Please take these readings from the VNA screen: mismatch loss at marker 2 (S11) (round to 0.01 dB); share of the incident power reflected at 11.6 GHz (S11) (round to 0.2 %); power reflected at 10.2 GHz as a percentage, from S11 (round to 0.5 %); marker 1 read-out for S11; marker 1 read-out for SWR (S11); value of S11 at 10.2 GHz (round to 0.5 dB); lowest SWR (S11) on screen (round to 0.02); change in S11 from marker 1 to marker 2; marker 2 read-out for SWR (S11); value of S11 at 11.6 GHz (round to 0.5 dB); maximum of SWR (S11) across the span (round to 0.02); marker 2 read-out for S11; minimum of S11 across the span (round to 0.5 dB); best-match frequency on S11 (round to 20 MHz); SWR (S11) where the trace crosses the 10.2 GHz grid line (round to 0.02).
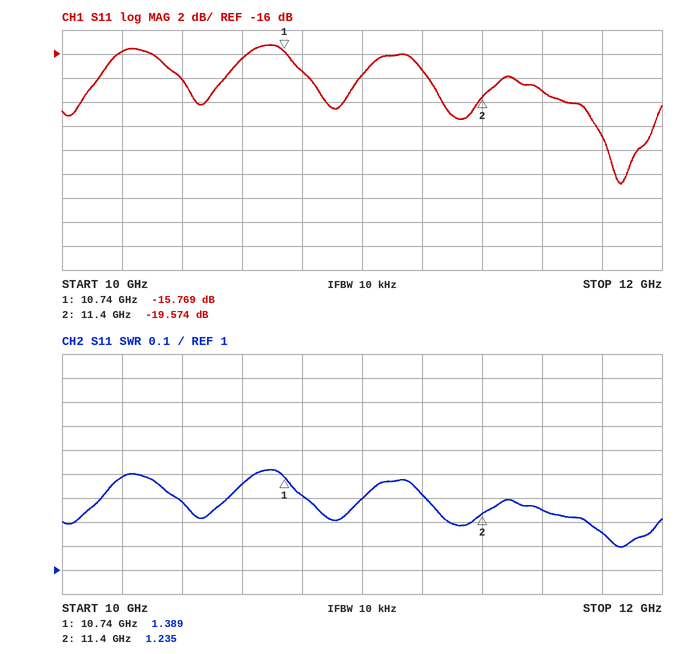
0.05 dB
1.2 %
2.5 %
-15.769 dB
1.389
-16.0 dB
1.10
-3.805 dB
1.235
-19.0 dB
1.42
-19.574 dB
-27.0 dB
11.86 GHz
1.38
